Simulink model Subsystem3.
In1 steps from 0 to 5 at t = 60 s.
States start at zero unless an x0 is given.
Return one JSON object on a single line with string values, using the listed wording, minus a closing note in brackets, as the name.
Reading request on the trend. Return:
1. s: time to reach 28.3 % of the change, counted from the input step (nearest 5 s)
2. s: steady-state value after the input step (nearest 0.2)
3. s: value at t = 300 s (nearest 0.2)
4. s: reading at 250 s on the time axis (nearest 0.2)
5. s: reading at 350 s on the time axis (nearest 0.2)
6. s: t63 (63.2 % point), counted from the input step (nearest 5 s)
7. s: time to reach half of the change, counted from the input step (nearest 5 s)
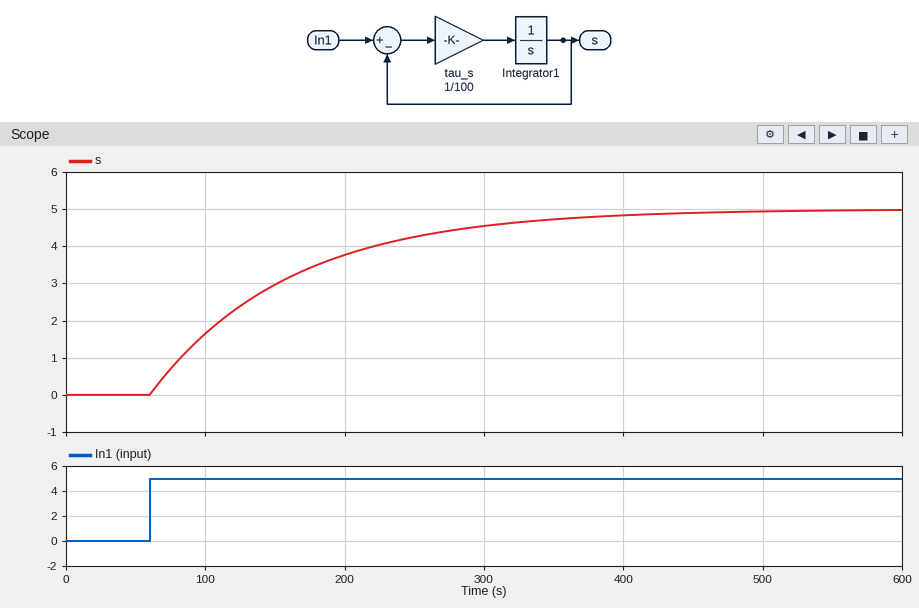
{"s: time to reach 28.3 % of the change, counted from the input step": "35 s", "s: steady-state value after the input step": "5.0", "s: value at t = 300 s": "4.6", "s: reading at 250 s on the time axis": "4.2", "s: reading at 350 s on the time axis": "4.8", "s: t63 (63.2 % point), counted from the input step": "100 s", "s: time to reach half of the change, counted from the input step": "70 s"}
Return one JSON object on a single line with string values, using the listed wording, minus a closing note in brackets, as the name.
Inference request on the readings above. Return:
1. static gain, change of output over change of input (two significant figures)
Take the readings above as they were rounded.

{"static gain, change of output over change of input": "1.0"}
